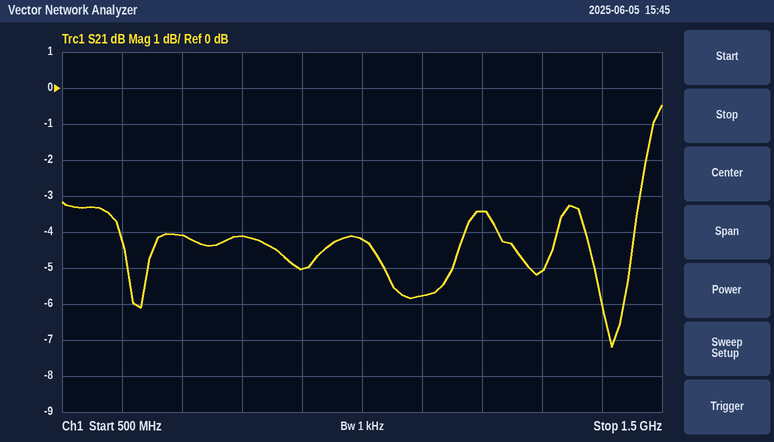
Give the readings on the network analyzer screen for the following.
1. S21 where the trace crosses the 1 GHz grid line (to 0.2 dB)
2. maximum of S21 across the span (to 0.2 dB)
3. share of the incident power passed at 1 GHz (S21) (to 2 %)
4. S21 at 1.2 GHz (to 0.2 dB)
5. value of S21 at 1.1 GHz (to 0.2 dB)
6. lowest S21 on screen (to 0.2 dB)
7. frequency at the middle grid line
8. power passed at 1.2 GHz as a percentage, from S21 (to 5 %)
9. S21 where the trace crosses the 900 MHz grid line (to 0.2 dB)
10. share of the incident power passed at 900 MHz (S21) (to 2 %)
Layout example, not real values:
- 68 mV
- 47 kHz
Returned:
- -4.2 dB
- -0.4 dB
- 38 %
- -3.4 dB
- -5.8 dB
- -7.2 dB
- 1 GHz
- 45 %
- -5.0 dB
- 32 %
